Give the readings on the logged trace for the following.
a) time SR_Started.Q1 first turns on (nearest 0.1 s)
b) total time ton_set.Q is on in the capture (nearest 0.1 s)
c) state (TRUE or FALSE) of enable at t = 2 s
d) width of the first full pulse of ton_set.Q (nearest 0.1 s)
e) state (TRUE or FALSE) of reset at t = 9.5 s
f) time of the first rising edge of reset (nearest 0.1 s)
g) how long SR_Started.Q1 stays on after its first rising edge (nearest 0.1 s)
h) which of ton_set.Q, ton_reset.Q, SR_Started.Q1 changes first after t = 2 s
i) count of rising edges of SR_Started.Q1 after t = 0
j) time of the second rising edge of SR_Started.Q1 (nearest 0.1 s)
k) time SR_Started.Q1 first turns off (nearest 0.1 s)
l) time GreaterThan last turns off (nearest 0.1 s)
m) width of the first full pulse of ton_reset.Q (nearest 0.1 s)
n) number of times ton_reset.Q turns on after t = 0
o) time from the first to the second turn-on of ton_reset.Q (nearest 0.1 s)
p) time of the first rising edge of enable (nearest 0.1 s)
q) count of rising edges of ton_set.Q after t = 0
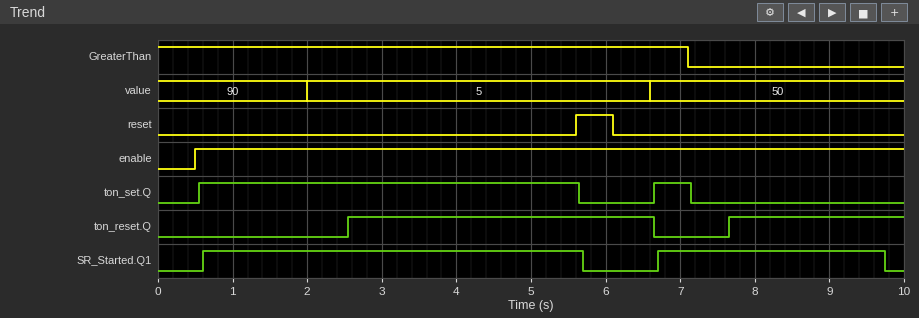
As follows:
0.6 s
5.6 s
TRUE
5.1 s
FALSE
5.6 s
5.1 s
ton_reset.Q
2
6.7 s
5.7 s
7.1 s
4.1 s
2
5.1 s
0.5 s
2
